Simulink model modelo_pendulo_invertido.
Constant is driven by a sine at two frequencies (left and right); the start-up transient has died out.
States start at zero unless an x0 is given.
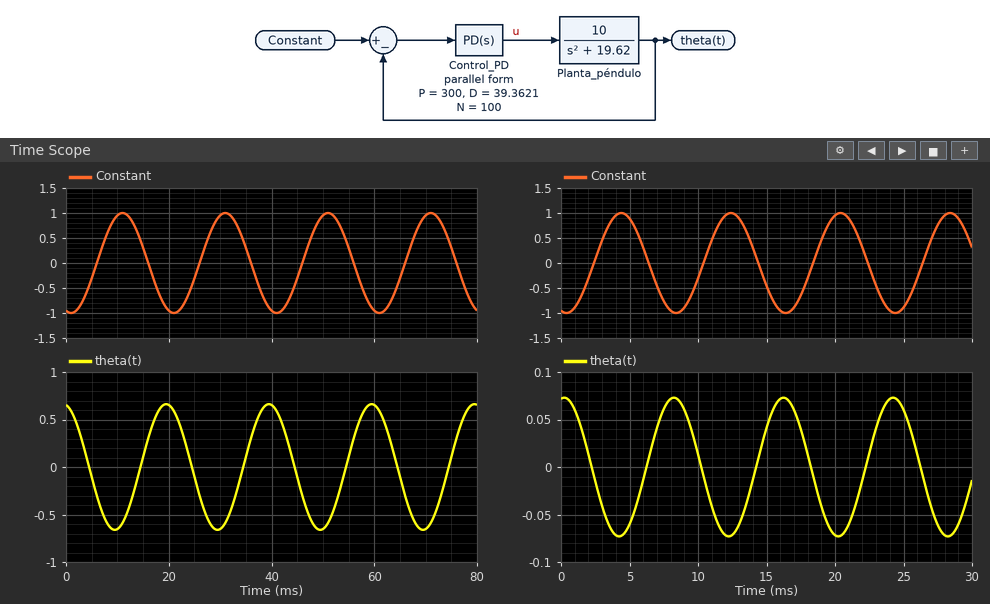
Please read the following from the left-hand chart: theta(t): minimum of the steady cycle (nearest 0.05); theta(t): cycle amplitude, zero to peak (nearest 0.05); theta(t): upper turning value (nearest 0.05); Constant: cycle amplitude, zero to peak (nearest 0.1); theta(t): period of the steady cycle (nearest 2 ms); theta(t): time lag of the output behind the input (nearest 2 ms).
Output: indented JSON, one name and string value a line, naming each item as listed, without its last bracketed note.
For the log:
{
  "theta(t): minimum of the steady cycle": "-0.65",
  "theta(t): cycle amplitude, zero to peak": "0.65",
  "theta(t): upper turning value": "0.65",
  "Constant: cycle amplitude, zero to peak": "1.0",
  "theta(t): period of the steady cycle": "20 ms",
  "theta(t): time lag of the output behind the input": "8 ms"
}
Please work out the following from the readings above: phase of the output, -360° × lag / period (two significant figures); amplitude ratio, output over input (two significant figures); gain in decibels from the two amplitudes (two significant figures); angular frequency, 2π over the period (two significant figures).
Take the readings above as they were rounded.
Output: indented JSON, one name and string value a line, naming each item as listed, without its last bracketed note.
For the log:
{
  "phase of the output, -360° × lag / period": "-140°",
  "amplitude ratio, output over input": "0.65",
  "gain in decibels from the two amplitudes": "-3.7 dB",
  "angular frequency, 2π over the period": "0.31 rad/ms"
}
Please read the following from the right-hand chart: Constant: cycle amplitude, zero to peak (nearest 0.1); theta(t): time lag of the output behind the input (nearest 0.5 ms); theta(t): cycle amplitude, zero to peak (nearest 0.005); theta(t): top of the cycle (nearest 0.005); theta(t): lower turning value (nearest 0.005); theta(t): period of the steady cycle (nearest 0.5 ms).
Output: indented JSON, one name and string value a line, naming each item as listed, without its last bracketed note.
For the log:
{
  "Constant: cycle amplitude, zero to peak": "1.0",
  "theta(t): time lag of the output behind the input": "4.0 ms",
  "theta(t): cycle amplitude, zero to peak": "0.075",
  "theta(t): top of the cycle": "0.075",
  "theta(t): lower turning value": "-0.075",
  "theta(t): period of the steady cycle": "8.0 ms"
}
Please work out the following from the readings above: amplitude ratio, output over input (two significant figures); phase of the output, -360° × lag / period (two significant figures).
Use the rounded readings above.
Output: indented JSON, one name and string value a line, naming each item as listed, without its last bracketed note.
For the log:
{
  "amplitude ratio, output over input": "0.075",
  "phase of the output, -360° × lag / period": "-180°"
}
